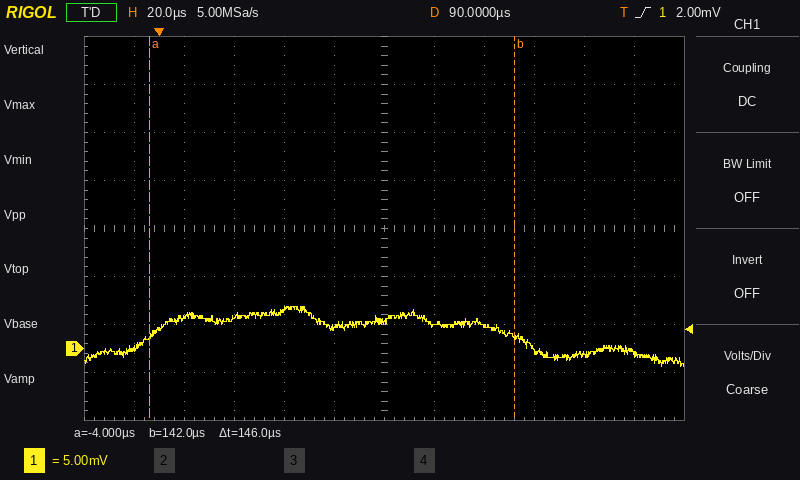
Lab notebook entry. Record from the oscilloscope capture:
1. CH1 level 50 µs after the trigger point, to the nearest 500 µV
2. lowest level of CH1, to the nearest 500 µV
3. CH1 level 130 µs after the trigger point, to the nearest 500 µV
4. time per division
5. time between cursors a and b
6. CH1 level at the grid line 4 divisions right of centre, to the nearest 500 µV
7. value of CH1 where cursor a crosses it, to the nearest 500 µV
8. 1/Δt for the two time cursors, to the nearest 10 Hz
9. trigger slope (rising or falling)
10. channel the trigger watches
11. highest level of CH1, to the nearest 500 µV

4.0 mV
-2.0 mV
2.5 mV
20 µs
146 µs
-500 µV
1.5 mV
6.85 kHz
rising
CH1
4.5 mV
